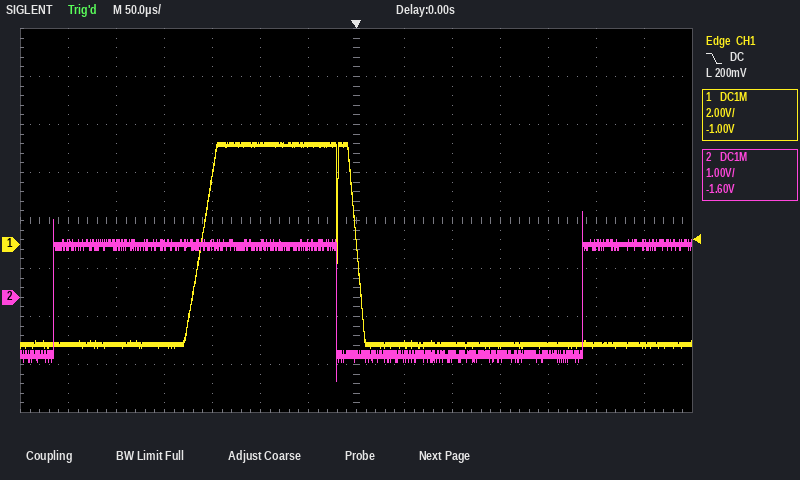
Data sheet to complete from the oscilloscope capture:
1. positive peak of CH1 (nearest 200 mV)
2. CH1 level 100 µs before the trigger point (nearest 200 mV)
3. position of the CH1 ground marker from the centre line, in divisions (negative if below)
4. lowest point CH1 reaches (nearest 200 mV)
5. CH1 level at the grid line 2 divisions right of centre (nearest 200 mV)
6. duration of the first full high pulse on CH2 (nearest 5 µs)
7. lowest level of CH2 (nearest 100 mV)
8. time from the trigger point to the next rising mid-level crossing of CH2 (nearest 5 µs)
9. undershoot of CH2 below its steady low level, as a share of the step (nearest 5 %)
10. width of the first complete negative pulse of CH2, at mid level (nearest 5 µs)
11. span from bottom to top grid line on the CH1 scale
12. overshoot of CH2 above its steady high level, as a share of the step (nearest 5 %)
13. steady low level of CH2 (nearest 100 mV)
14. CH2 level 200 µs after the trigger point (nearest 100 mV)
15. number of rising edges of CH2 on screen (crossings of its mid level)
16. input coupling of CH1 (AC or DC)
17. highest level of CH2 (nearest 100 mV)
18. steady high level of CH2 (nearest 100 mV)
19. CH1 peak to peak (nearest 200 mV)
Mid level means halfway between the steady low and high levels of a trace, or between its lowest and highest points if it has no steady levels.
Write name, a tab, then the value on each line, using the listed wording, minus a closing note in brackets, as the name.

positive peak of CH1	4.2 V
CH1 level 100 µs before the trigger point	4.2 V
position of the CH1 ground marker from the centre line, in divisions	-0.5 div
lowest point CH1 reaches	-4.4 V
CH1 level at the grid line 2 divisions right of centre	-4.2 V
duration of the first full high pulse on CH2	295 µs
lowest level of CH2	-1.8 V
time from the trigger point to the next rising mid-level crossing of CH2	235 µs
undershoot of CH2 below its steady low level, as a share of the step	25 %
width of the first complete negative pulse of CH2, at mid level	255 µs
span from bottom to top grid line on the CH1 scale	16 V
overshoot of CH2 above its steady high level, as a share of the step	30 %
steady low level of CH2	-1.2 V
CH2 level 200 µs after the trigger point	-1.2 V
number of rising edges of CH2 on screen	2
input coupling of CH1	DC
highest level of CH2	1.8 V
steady high level of CH2	1.1 V
CH1 peak to peak	8.6 V
